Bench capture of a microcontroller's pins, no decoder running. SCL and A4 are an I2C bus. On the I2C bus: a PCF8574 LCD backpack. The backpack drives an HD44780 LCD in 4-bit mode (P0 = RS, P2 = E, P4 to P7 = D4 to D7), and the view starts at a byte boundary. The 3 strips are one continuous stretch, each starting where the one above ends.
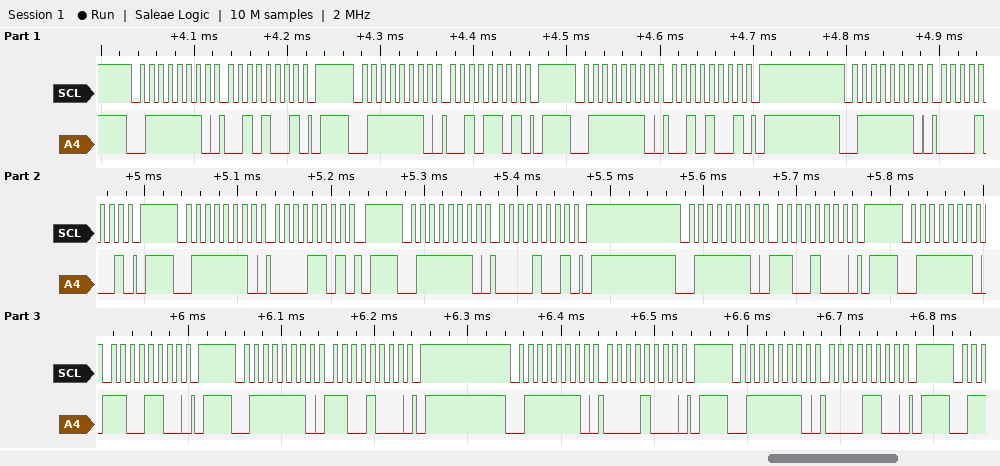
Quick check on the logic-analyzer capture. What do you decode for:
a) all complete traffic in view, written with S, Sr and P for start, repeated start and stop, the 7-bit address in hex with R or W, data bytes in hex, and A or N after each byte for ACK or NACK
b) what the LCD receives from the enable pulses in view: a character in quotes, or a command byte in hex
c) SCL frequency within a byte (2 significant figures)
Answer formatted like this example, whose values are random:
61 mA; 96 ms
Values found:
S 3FW A 29 A P S 3FW A 2D A P S 3FW A 29 A P S 3FW A 09 A P S 3FW A 0D A P S 3FW A 09 A P S 3FW A C8 A P S 3FW A CC A P S 3FW A C8 A P S 3FW A 08 A P S 3FW A 0C A P; ' '; 100 kHz
